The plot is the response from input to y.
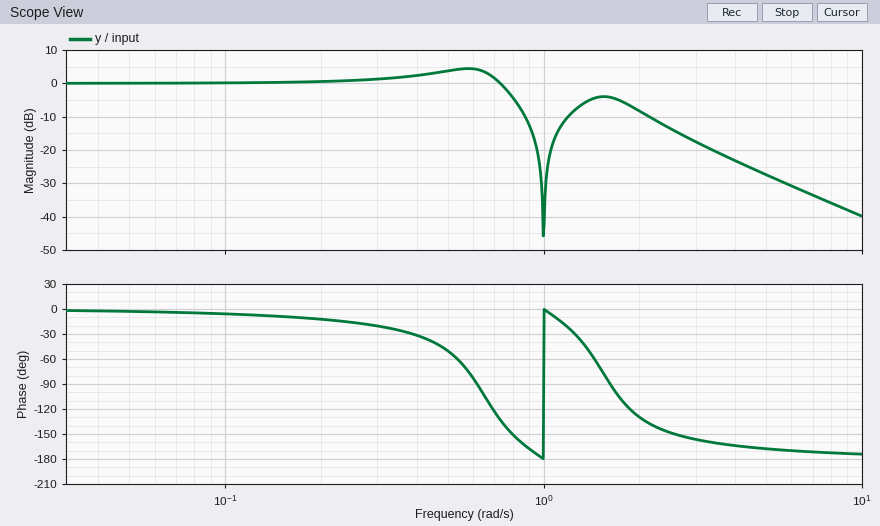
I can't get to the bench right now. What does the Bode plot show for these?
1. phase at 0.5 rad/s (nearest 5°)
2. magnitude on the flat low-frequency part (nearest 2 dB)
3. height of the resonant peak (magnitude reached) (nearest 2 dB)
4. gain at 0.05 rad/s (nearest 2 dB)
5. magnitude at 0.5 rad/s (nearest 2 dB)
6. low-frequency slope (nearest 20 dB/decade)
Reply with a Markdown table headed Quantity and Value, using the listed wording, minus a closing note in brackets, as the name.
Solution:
| Quantity | Value |
|---|---|
| phase at 0.5 rad/s | -50° |
| magnitude on the flat low-frequency part | 0 dB |
| height of the resonant peak (magnitude reached) | 4 dB |
| gain at 0.05 rad/s | 0 dB |
| magnitude at 0.5 rad/s | 4 dB |
| low-frequency slope | 0 dB/decade |
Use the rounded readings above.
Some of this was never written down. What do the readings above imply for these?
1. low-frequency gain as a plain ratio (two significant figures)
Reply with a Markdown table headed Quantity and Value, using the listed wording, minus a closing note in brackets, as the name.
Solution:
| Quantity | Value |
|---|---|
| low-frequency gain as a plain ratio | 1.0 |
